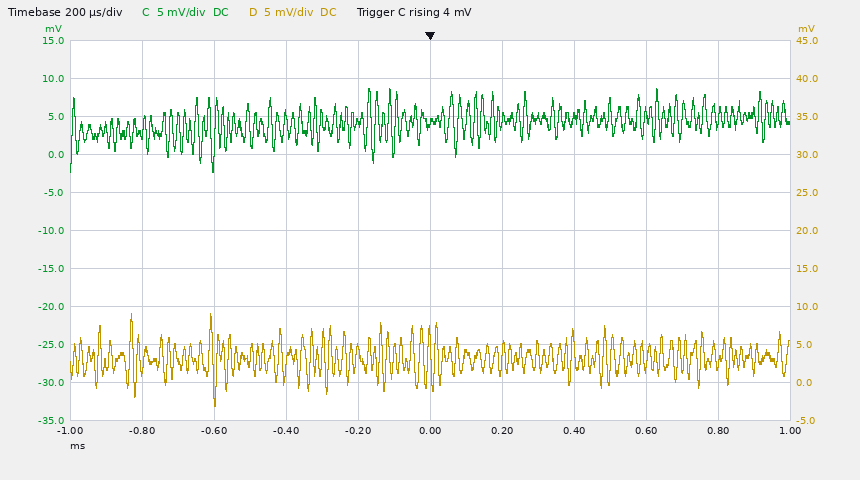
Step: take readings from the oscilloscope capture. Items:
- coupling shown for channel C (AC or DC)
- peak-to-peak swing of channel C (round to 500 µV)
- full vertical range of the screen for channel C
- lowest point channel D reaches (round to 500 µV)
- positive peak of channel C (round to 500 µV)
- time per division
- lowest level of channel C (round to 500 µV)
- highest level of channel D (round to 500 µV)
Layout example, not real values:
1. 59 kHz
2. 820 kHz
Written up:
1. DC
2. 11.0 mV
3. 50 mV
4. -3.0 mV
5. 8.5 mV
6. 200 µs
7. -2.5 mV
8. 9.0 mV
